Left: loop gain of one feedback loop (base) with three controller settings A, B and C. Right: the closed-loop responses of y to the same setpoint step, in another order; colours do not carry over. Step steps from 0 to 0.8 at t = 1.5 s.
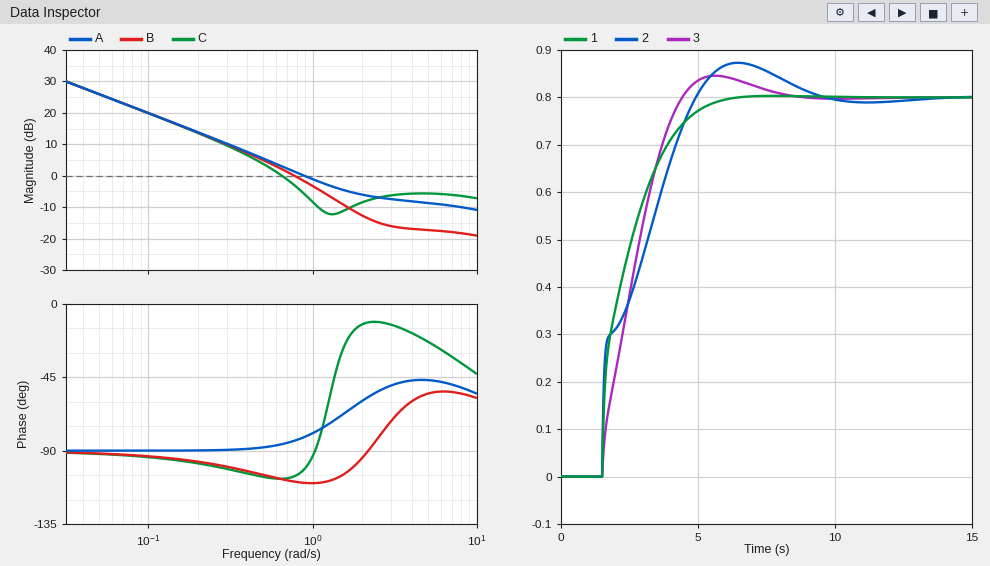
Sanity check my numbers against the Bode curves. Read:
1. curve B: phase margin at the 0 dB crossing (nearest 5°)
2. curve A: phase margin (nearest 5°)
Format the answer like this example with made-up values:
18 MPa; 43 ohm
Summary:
70°; 100°
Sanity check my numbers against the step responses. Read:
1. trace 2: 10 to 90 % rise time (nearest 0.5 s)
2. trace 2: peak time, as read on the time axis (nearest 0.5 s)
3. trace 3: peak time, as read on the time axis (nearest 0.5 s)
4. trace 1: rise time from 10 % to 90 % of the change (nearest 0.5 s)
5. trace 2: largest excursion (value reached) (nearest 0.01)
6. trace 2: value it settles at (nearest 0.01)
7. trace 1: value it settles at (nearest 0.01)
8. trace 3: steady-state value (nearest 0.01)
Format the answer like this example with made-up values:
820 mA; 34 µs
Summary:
3.0 s; 6.5 s; 5.5 s; 2.5 s; 0.87; 0.80; 0.80; 0.80
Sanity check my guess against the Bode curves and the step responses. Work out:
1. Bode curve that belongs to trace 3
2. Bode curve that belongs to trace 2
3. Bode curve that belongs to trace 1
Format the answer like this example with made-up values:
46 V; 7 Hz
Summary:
B; C; A
